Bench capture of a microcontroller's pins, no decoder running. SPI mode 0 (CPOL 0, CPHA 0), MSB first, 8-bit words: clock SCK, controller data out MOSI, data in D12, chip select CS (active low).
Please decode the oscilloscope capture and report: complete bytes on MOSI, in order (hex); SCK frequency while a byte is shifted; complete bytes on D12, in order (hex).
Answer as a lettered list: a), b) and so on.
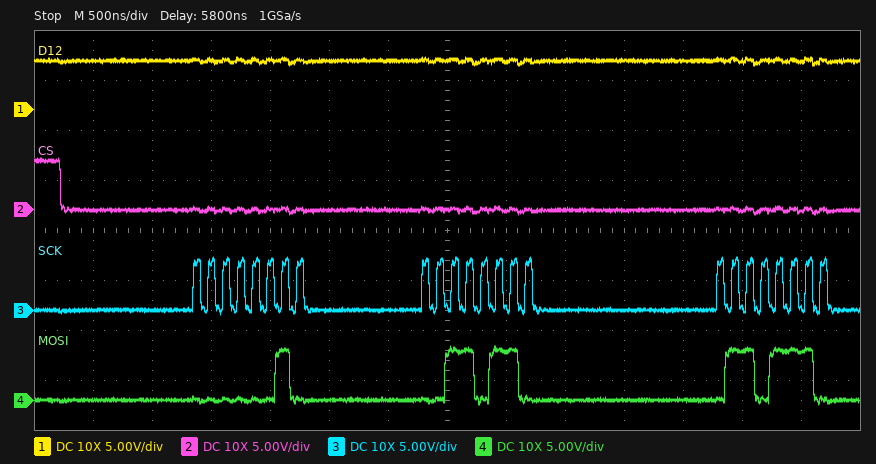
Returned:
a) 0x02 0x36 0x6E
b) 8 MHz
c) 0xFF 0xFF 0xFF
